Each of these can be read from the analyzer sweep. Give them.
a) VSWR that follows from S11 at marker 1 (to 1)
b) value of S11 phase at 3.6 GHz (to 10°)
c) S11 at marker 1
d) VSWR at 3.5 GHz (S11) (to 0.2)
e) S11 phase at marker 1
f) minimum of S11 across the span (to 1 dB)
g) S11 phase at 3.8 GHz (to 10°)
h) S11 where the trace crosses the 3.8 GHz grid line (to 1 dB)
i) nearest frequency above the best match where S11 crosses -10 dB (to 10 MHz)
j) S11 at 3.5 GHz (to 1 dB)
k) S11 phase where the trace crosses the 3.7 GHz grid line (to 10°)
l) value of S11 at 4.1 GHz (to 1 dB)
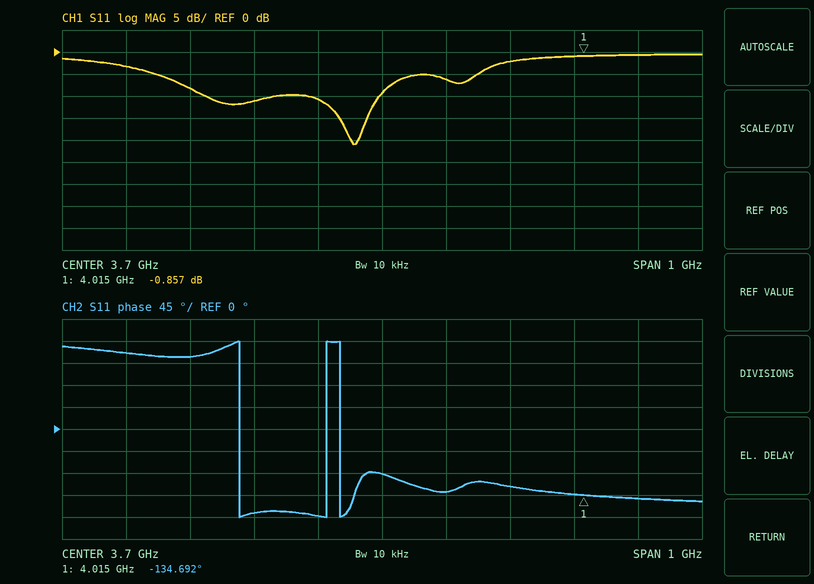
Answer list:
20
-180°
-0.857 dB
1.8
-134.692°
-21 dB
-130°
-6 dB
3.70 GHz
-11 dB
-90°
-1 dB
